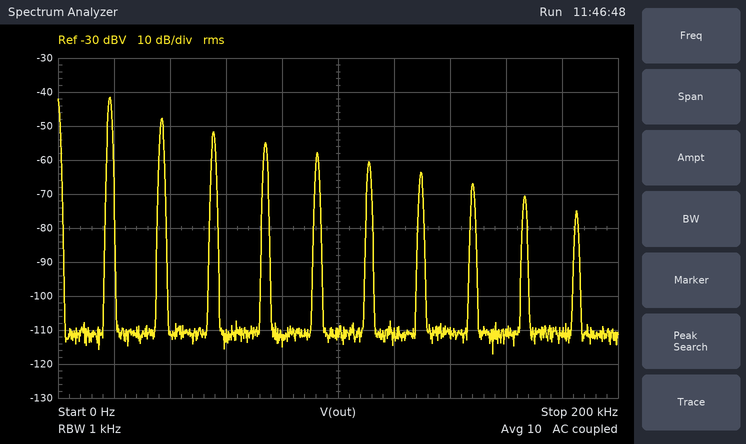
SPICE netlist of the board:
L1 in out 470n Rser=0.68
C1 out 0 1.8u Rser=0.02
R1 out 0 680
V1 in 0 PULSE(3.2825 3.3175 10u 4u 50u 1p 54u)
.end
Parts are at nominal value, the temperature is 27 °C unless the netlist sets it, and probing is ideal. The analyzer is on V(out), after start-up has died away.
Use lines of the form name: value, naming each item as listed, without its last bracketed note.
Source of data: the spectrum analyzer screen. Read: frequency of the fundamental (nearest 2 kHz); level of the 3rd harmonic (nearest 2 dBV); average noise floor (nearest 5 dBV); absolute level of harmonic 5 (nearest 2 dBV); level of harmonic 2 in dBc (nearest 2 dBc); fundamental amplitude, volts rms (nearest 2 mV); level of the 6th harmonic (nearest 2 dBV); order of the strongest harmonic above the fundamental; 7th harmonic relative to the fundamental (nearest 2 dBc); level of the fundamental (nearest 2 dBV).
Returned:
frequency of the fundamental: 18 kHz
level of the 3rd harmonic: -52 dBV
average noise floor: -110 dBV
absolute level of harmonic 5: -58 dBV
level of harmonic 2 in dBc: -6 dBc
fundamental amplitude, volts rms: 8 mV
level of the 6th harmonic: -60 dBV
order of the strongest harmonic above the fundamental: 2
7th harmonic relative to the fundamental: -22 dBc
level of the fundamental: -42 dBV
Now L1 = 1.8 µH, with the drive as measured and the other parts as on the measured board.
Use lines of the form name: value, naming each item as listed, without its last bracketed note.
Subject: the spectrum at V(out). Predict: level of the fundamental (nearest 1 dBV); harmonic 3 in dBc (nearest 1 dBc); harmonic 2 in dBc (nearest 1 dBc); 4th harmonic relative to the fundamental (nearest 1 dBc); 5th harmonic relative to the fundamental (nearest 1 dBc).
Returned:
level of the fundamental: -41 dBV
harmonic 3 in dBc: -8 dBc
harmonic 2 in dBc: -5 dBc
4th harmonic relative to the fundamental: -10 dBc
5th harmonic relative to the fundamental: -14 dBc
